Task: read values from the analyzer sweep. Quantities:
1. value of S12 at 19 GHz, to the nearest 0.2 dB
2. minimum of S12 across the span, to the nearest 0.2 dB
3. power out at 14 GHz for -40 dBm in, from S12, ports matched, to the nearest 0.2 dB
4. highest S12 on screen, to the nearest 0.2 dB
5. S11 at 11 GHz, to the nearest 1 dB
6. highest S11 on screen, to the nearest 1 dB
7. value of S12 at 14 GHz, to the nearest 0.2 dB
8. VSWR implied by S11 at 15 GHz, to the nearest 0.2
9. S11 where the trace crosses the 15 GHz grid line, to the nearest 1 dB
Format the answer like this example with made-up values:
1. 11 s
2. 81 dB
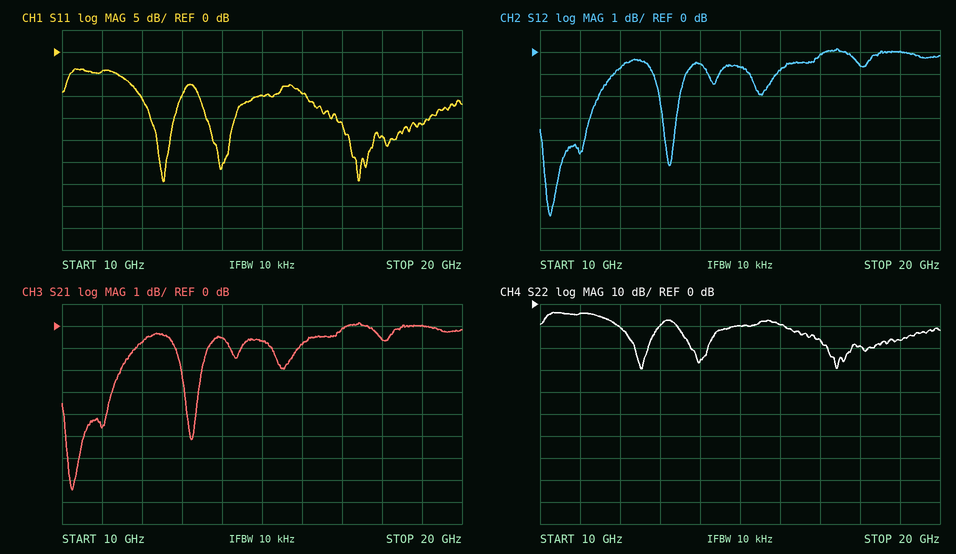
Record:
1. 0.0 dB
2. -7.4 dB
3. -40.6 dBm
4. 0.2 dB
5. -4 dB
6. -4 dB
7. -0.6 dB
8. 2.0
9. -10 dB
